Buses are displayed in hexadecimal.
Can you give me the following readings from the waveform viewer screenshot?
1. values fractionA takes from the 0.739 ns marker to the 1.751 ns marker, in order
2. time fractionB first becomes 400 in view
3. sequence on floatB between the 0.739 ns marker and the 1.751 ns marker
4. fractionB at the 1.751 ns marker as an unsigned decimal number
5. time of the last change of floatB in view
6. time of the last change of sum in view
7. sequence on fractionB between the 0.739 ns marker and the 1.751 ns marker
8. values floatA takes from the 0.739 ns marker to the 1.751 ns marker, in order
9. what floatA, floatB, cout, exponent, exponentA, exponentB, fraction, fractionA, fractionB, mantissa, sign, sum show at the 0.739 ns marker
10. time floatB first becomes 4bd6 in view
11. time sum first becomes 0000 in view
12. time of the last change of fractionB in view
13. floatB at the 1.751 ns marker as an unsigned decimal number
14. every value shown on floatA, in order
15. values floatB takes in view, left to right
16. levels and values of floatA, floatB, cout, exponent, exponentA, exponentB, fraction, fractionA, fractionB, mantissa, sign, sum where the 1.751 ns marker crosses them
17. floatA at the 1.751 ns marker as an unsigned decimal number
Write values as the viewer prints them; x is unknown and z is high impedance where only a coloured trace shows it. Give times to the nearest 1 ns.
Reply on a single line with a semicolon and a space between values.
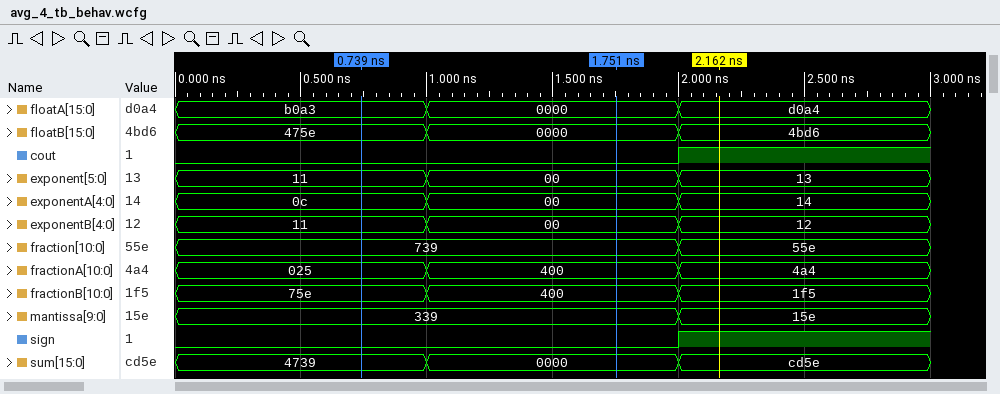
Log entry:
025, 400; 1 ns; 475e, 0000; 1024; 2 ns; 2 ns; 75e, 400; b0a3, 0000; floatA=b0a3, floatB=475e, cout=0, exponent=11, exponentA=0c, exponentB=11, fraction=739, fractionA=025, fractionB=75e, mantissa=339, sign=0, sum=4739; 2 ns; 1 ns; 2 ns; 0; b0a3, 0000, d0a4; 475e, 0000, 4bd6; floatA=0000, floatB=0000, cout=0, exponent=00, exponentA=00, exponentB=00, fraction=739, fractionA=400, fractionB=400, mantissa=339, sign=0, sum=0000; 0
